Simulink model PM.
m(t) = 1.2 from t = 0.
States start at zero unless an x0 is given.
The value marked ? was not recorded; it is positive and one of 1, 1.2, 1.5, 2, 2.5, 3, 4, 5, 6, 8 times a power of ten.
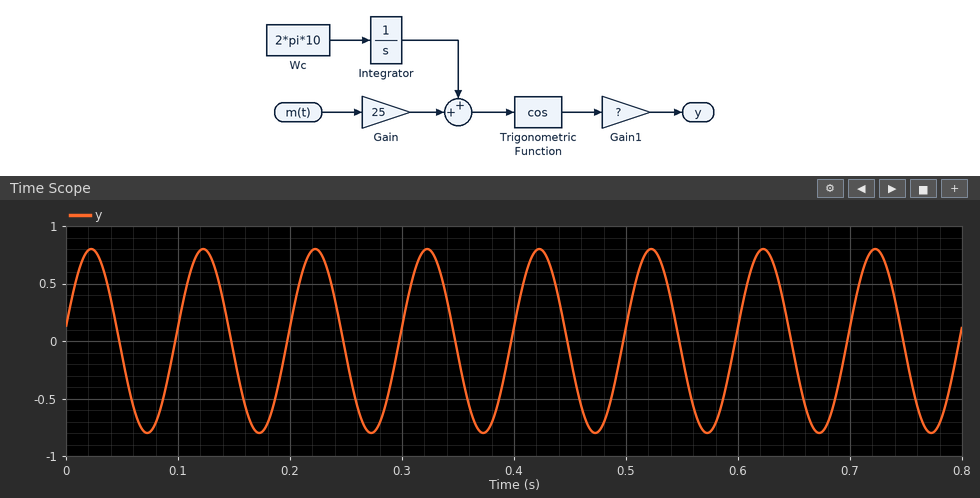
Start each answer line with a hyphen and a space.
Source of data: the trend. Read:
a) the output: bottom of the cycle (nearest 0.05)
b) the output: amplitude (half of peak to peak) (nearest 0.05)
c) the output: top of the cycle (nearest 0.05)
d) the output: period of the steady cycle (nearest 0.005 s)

- -0.80
- 0.80
- 0.80
- 0.100 s
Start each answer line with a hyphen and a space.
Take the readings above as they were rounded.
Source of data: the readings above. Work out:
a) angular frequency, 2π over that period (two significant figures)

- 63 rad/s
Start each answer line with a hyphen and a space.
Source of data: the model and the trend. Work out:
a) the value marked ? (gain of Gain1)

- 0.8
